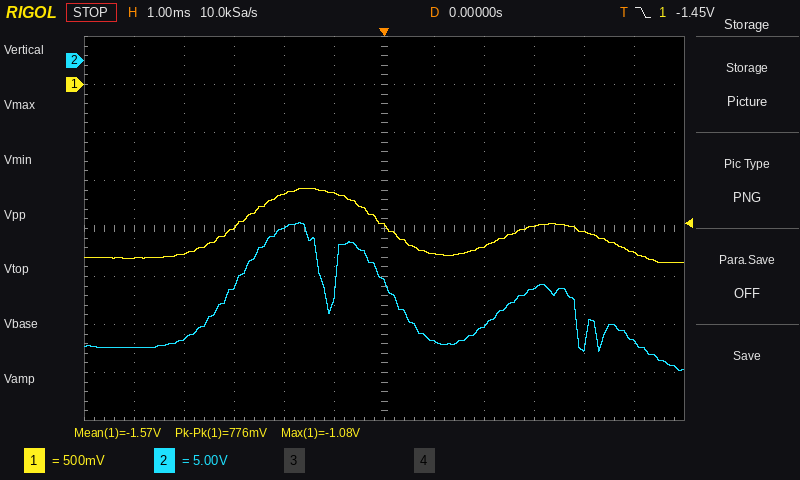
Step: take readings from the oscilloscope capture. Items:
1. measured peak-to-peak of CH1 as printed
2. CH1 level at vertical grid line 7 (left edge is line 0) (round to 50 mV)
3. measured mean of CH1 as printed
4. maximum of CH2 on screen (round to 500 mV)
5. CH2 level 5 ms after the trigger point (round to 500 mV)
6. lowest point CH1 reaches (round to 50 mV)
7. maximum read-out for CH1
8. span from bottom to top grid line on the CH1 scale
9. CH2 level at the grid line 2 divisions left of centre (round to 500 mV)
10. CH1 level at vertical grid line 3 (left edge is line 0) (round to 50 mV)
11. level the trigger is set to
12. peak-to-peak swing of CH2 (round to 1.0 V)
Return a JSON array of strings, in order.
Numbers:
["776 mV", "-1.75 V", "-1.57 V", "-17.0 V", "-29.5 V", "-1.85 V", "-1.08 V", "4 V", "-17.5 V", "-1.50 V", "-1.45 V", "15.0 V"]
